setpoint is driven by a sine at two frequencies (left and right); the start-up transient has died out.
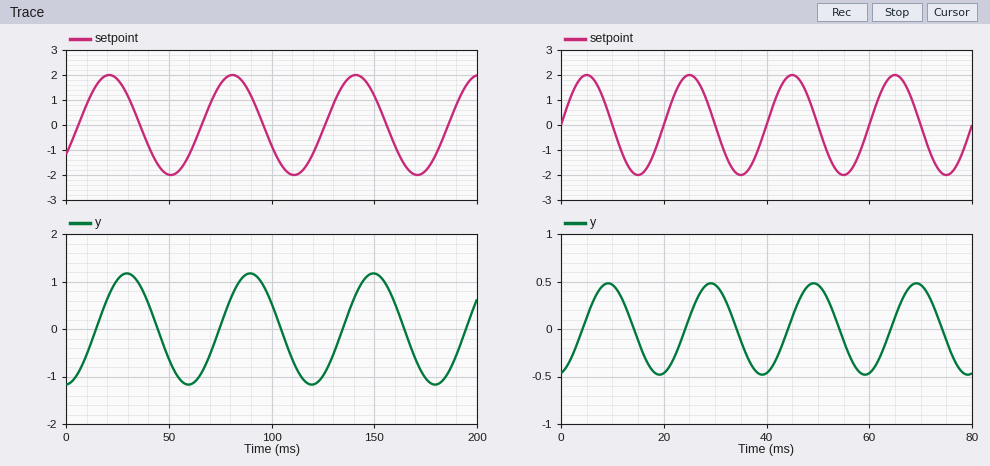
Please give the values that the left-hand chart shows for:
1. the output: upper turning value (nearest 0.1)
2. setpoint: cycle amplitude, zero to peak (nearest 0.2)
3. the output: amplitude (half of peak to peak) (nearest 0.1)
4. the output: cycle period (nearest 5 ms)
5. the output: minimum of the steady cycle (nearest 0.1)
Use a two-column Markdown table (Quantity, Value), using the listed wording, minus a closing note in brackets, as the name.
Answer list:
| Quantity | Value |
|---|---|
| the output: upper turning value | 1.2 |
| setpoint: cycle amplitude, zero to peak | 2.0 |
| the output: amplitude (half of peak to peak) | 1.2 |
| the output: cycle period | 60 ms |
| the output: minimum of the steady cycle | -1.2 |
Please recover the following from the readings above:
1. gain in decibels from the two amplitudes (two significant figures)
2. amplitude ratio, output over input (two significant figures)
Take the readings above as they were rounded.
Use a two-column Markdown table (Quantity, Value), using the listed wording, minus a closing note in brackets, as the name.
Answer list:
| Quantity | Value |
|---|---|
| gain in decibels from the two amplitudes | -4.4 dB |
| amplitude ratio, output over input | 0.60 |
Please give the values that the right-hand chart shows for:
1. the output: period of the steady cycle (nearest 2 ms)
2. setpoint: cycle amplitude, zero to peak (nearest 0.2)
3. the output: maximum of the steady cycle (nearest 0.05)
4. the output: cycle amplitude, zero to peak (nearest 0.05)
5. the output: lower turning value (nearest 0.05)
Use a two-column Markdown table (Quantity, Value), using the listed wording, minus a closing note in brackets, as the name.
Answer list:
| Quantity | Value |
|---|---|
| the output: period of the steady cycle | 20 ms |
| setpoint: cycle amplitude, zero to peak | 2.0 |
| the output: maximum of the steady cycle | 0.50 |
| the output: cycle amplitude, zero to peak | 0.50 |
| the output: lower turning value | -0.50 |
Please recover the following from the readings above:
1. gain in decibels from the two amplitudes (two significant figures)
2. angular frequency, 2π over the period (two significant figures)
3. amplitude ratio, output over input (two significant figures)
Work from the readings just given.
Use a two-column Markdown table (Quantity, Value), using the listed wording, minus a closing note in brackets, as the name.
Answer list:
| Quantity | Value |
|---|---|
| gain in decibels from the two amplitudes | -12 dB |
| angular frequency, 2π over the period | 0.31 rad/ms |
| amplitude ratio, output over input | 0.25 |
